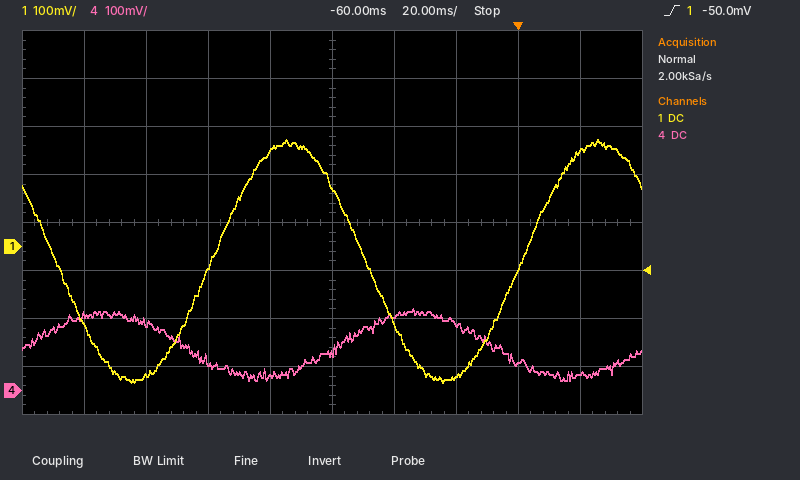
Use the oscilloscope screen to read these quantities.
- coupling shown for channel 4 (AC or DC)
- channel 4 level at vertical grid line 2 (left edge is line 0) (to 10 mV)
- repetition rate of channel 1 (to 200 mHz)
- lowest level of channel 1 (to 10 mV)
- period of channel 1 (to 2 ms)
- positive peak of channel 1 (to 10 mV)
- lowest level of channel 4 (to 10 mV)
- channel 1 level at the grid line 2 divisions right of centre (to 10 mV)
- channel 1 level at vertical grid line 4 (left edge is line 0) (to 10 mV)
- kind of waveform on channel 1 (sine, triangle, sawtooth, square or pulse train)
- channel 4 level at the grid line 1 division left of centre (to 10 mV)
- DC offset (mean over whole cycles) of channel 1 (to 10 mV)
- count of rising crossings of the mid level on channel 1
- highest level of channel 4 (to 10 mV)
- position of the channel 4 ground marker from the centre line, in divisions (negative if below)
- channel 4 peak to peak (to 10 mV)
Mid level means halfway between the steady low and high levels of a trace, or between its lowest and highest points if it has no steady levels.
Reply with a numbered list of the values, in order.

1. DC
2. 140 mV
3. 10.0 Hz
4. -280 mV
5. 100 ms
6. 220 mV
7. 20 mV
8. -270 mV
9. 200 mV
10. sine
11. 30 mV
12. -30 mV
13. 2
14. 170 mV
15. -3.5 div
16. 150 mV
